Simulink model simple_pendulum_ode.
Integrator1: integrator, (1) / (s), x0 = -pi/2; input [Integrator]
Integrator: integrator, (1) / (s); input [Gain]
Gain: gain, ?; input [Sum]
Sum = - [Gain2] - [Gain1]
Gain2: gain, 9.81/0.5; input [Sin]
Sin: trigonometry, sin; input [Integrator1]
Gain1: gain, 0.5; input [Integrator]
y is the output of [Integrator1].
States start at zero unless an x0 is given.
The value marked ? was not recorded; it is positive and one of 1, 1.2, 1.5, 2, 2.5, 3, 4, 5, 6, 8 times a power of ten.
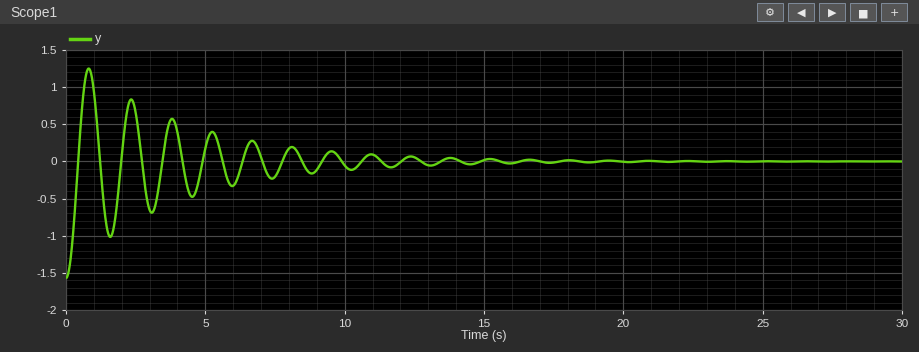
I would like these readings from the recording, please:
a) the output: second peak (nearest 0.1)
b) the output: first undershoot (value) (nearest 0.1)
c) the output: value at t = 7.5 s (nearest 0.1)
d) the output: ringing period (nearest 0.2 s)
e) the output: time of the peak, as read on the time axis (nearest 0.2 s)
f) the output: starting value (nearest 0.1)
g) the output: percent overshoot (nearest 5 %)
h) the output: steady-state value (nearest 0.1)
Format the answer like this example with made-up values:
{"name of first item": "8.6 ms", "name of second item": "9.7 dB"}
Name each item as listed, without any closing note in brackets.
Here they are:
{"the output: second peak": "0.8", "the output: first undershoot (value)": "-1.0", "the output: value at t = 7.5 s": "-0.2", "the output: ringing period": "1.6 s", "the output: time of the peak, as read on the time axis": "0.8 s", "the output: starting value": "-1.6", "the output: percent overshoot": "80 %", "the output: steady-state value": "0.0"}
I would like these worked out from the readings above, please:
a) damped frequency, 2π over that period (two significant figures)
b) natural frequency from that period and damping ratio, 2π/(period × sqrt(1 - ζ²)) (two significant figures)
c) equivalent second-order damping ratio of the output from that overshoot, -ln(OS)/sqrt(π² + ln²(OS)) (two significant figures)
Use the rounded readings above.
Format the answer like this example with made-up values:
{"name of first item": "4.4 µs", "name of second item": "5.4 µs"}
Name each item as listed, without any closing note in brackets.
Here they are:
{"damped frequency, 2π over that period": "3.9 rad/s", "natural frequency from that period and damping ratio, 2π/(period × sqrt(1 - ζ²))": "3.9 rad/s", "equivalent second-order damping ratio of the output from that overshoot, -ln(OS)/sqrt(π² + ln²(OS))": "0.071"}
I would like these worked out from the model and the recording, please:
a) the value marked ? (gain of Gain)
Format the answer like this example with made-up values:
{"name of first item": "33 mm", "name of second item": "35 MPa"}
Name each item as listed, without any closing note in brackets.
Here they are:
{"the value marked ?": "1"}
